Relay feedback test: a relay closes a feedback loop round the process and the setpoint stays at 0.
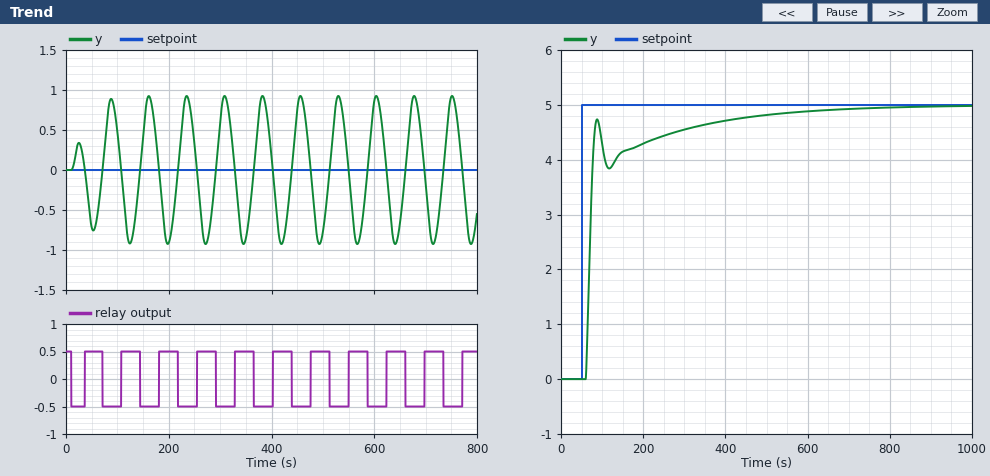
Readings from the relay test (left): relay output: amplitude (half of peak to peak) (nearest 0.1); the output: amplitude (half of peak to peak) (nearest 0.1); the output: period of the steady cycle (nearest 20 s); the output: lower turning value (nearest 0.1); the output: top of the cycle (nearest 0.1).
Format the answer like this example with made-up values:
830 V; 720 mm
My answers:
0.5; 0.9; 80 s; -0.9; 0.9
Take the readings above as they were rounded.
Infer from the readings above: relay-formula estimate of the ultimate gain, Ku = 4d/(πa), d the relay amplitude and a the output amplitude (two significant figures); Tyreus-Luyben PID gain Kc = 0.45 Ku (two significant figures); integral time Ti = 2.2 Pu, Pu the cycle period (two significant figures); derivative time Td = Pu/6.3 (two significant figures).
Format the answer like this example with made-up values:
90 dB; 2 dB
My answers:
0.71; 0.32; 180 s; 13 s
